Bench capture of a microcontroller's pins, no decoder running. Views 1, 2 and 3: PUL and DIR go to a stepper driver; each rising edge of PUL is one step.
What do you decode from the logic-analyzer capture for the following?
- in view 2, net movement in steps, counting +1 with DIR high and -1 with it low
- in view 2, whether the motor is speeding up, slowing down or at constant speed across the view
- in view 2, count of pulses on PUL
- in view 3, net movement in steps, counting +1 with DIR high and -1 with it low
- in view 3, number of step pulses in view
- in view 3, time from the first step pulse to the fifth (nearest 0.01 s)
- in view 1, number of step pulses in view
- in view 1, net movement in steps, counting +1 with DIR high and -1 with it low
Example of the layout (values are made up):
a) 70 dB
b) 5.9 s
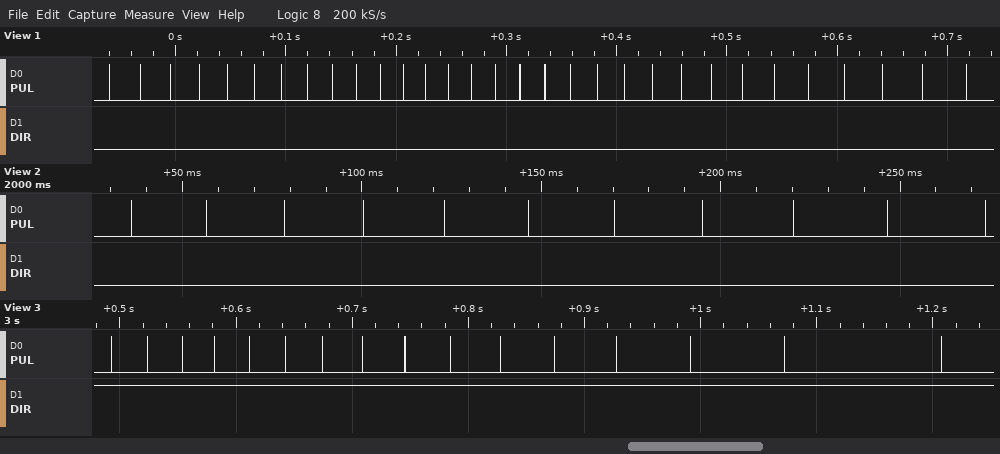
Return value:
a) -11
b) slowing down
c) 11
d) +16
e) 16
f) 0.12 s
g) 31
h) -31
